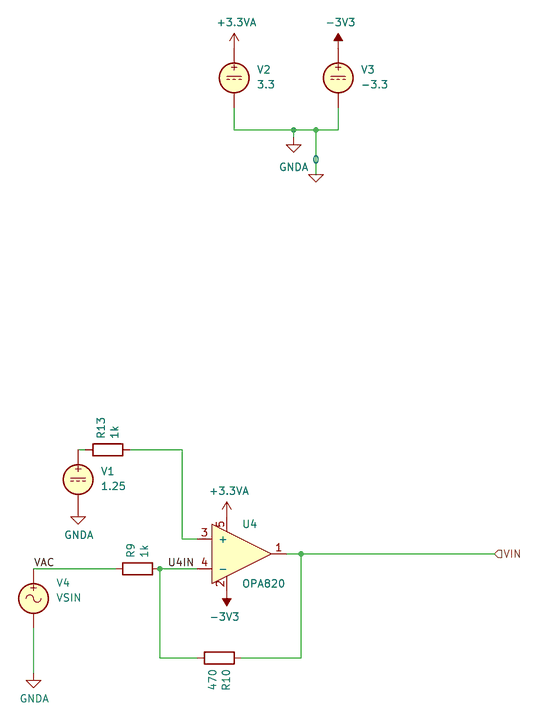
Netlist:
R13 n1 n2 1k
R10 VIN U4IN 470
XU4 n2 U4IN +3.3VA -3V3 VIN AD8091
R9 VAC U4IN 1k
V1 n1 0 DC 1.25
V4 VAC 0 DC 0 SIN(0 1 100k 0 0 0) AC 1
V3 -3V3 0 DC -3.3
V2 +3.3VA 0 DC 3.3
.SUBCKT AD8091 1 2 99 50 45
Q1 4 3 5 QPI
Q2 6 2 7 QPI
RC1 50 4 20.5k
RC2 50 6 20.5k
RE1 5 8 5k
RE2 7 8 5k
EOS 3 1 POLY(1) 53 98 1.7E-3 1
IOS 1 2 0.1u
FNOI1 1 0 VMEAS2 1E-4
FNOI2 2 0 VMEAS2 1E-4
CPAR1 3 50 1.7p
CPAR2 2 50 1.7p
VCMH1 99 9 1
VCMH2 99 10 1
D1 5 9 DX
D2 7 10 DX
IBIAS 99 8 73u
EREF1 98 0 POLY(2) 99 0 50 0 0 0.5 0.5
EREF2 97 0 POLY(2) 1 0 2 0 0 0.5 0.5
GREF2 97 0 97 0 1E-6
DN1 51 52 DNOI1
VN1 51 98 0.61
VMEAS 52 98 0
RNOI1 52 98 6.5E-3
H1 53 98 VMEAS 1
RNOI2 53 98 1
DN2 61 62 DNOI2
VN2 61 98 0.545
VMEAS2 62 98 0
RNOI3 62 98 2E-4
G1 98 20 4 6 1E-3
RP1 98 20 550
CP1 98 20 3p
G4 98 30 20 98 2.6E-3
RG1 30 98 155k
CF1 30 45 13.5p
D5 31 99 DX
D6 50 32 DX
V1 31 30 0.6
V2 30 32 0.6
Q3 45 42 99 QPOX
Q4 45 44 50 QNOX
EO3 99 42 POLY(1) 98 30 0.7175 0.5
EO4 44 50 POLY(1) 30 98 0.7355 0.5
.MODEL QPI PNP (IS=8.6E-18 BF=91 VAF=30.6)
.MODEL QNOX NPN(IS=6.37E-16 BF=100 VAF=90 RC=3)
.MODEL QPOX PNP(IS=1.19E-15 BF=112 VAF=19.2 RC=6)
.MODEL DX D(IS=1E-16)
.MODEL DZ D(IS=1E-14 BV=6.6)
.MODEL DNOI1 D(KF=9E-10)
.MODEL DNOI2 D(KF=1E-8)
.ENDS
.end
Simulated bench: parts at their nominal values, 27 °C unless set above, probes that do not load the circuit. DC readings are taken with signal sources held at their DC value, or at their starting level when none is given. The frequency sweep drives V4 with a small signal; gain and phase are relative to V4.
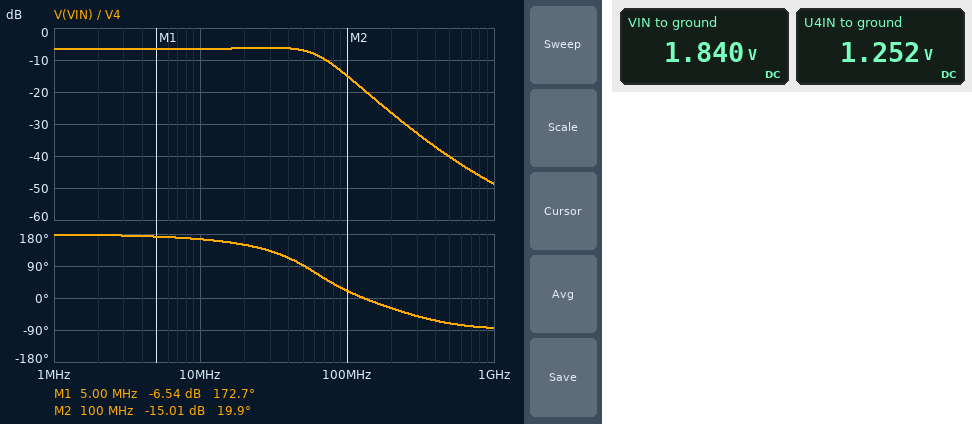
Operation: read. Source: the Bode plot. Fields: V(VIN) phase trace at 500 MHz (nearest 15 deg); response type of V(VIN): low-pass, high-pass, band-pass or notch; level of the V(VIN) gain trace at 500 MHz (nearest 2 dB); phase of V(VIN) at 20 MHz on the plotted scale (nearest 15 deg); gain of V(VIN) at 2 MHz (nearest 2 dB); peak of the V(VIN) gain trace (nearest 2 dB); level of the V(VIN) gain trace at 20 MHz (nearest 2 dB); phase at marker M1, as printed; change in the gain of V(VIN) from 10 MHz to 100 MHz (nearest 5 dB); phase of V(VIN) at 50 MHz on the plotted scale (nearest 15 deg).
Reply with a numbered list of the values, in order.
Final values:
1. -75 deg
2. low-pass
3. -40 dB
4. 150 deg
5. -6 dB
6. -6 dB
7. -6 dB
8. 172.7 deg
9. -10 dB
10. 90 deg
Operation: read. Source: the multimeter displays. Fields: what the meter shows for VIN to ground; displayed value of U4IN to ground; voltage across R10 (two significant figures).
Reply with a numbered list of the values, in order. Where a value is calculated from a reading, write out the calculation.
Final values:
1. 1.840 V
2. 1.252 V
3. 1.84 V - 1.252 V = 590 mV
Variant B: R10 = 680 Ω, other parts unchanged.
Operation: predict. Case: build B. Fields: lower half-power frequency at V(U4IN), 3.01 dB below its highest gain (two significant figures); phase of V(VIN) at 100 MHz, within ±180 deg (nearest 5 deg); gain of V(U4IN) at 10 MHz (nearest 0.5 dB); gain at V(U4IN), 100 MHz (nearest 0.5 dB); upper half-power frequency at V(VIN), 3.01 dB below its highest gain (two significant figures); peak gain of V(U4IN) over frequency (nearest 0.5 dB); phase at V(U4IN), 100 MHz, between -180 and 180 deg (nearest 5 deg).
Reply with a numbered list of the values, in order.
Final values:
1. 33 MHz
2. 15 deg
3. -18.5 dB
4. -6.5 dB
5. 59 MHz
6. -5.0 dB
7. -20 deg
